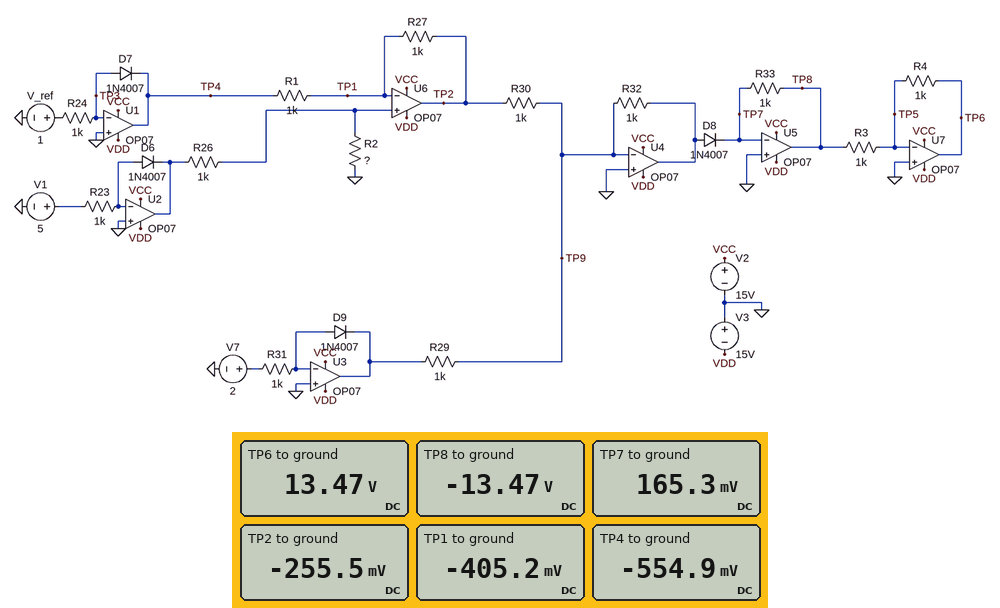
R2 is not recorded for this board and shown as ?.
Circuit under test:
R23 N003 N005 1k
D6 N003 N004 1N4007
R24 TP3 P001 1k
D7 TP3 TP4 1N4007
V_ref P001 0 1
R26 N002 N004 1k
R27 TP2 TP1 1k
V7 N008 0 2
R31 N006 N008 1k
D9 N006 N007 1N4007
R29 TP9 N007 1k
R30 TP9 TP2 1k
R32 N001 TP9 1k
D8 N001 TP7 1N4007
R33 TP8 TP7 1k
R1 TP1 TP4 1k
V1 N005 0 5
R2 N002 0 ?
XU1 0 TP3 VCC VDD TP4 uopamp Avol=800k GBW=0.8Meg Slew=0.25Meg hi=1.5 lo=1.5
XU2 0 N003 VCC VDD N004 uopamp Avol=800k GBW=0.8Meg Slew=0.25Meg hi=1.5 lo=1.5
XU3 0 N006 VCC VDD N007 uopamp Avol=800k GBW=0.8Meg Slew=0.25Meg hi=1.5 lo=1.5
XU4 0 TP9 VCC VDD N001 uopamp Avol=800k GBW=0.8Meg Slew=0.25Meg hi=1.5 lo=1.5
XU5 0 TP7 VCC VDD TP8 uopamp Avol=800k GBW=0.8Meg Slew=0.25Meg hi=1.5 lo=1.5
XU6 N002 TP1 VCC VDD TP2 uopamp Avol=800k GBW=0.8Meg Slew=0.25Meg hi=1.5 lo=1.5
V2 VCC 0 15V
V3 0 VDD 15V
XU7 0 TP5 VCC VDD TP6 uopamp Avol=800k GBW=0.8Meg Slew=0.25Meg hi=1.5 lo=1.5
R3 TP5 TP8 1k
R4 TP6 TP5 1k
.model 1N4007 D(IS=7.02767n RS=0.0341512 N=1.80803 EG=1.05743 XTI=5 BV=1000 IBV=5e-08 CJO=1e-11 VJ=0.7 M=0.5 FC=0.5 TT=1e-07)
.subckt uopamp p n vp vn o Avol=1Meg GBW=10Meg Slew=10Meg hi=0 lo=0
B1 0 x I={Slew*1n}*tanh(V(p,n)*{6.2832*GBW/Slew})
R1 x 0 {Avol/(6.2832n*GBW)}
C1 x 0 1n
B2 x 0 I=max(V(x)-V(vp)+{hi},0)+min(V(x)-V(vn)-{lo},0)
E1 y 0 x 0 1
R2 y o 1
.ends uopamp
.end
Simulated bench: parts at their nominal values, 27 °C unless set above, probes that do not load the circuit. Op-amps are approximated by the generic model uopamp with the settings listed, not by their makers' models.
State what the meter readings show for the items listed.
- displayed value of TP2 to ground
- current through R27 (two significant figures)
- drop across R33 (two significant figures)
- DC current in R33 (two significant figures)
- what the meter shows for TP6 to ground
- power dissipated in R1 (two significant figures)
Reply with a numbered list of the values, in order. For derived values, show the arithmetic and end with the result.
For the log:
1. -255.5 mV
2. (-255.5 mV - (-405.2 mV)) / 1 kΩ = 150 µA
3. 165.3 mV - (-13.47 V) = 14 V
4. (165.3 mV - (-13.47 V)) / 1 kΩ = 14 mA
5. 13.47 V
6. (-405.2 mV - (-554.9 mV))^2 / 1 kΩ = 22 µW
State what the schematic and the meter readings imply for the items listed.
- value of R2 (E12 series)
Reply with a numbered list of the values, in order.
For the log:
1. 1.8 kΩ
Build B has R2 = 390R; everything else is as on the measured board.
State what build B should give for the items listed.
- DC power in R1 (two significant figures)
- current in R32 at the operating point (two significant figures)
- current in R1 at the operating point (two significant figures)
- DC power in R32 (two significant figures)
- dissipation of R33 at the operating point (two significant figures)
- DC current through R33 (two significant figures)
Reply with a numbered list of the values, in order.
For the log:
1. 140 µW
2. 390 µA
3. 380 µA
4. 150 µW
5. 730 nW
6. 27 µA
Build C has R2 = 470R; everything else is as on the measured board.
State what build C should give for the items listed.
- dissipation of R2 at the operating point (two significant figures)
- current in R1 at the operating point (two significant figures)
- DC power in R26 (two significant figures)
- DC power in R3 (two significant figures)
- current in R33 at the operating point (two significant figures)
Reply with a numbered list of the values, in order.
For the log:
1. 86 µW
2. 350 µA
3. 180 µW
4. 6.1 µW
5. 78 µA
